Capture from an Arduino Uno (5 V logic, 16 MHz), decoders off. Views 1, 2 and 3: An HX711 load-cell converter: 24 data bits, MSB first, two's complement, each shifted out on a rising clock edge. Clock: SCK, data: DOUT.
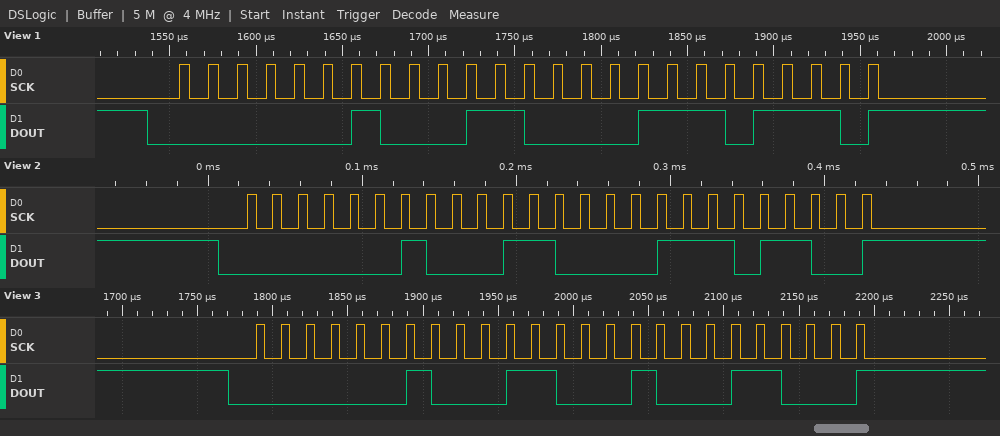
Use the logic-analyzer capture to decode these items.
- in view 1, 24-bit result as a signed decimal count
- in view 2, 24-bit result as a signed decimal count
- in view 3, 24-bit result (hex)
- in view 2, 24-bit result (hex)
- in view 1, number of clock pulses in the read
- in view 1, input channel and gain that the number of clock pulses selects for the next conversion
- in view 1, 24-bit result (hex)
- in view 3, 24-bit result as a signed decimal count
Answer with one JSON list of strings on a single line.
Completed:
["143598", "143596", "0x023118", "0x0230EC", "25", "channel A, gain 128", "0x0230EE", "143640"]
